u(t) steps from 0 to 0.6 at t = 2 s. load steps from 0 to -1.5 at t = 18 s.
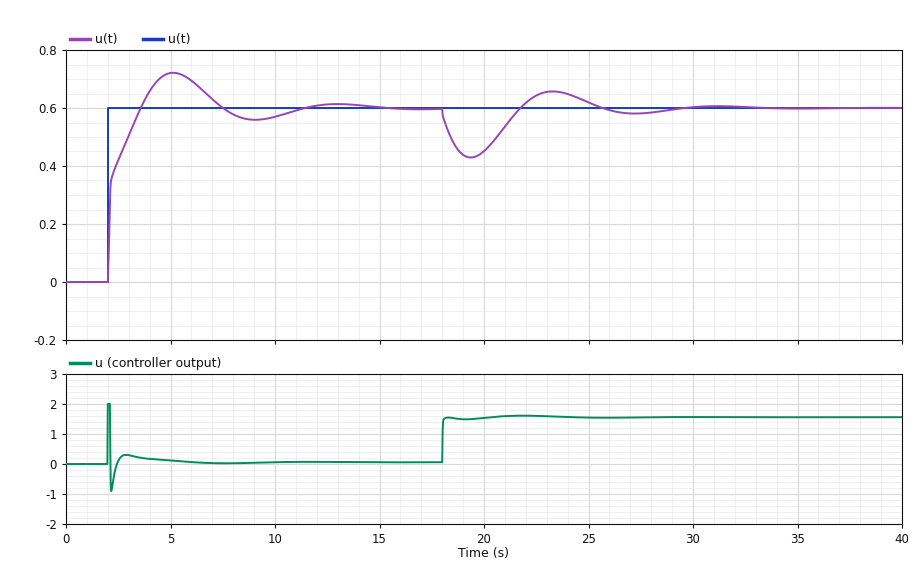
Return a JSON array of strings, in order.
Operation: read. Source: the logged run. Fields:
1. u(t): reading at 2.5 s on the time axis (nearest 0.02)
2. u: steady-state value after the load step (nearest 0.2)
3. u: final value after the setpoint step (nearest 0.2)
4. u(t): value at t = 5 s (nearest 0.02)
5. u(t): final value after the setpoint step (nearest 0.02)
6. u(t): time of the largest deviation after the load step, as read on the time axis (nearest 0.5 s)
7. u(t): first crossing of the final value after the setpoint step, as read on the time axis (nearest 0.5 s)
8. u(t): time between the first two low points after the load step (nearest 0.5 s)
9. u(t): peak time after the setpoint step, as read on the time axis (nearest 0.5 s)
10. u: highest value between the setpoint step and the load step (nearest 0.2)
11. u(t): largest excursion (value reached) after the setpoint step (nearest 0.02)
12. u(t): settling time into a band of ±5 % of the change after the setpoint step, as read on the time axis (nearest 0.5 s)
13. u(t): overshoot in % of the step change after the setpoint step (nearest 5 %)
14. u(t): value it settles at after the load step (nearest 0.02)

["0.42", "1.6", "0.0", "0.72", "0.60", "19.5 s", "3.5 s", "8.0 s", "5.0 s", "2.0", "0.72", "10.0 s", "20 %", "0.60"]
